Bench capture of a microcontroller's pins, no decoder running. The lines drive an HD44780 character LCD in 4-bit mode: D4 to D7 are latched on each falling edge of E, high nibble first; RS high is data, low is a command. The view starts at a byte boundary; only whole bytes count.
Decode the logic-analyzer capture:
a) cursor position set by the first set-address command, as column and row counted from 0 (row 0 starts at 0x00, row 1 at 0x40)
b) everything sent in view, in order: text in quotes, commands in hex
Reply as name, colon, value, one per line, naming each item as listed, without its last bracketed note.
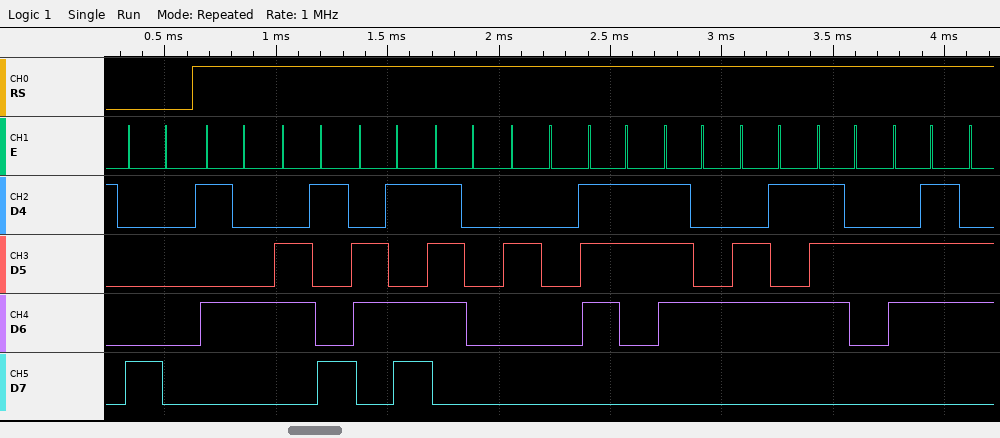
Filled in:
cursor position set by the first set-address command, as column and row counted from 0: column 0, row 0
everything sent in view, in order: text in quotes, commands in hex: 0x80 "Timp sterg"
